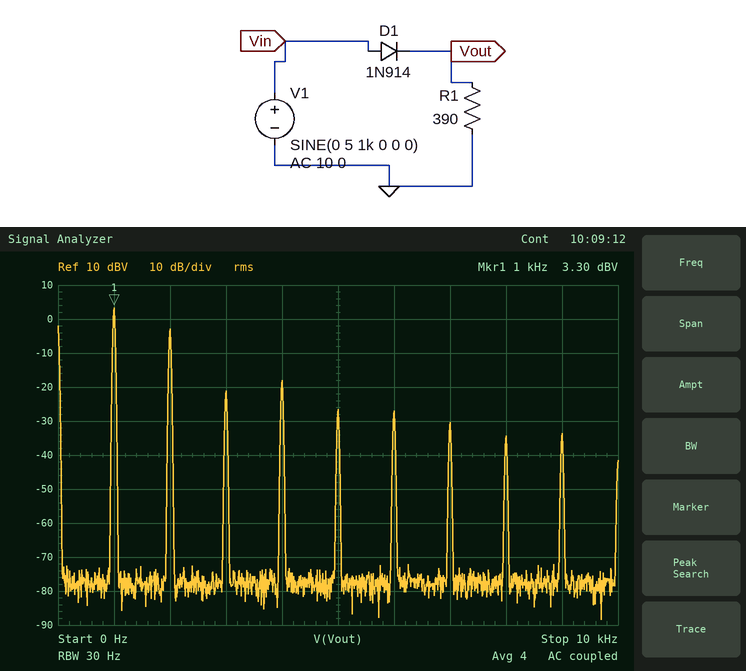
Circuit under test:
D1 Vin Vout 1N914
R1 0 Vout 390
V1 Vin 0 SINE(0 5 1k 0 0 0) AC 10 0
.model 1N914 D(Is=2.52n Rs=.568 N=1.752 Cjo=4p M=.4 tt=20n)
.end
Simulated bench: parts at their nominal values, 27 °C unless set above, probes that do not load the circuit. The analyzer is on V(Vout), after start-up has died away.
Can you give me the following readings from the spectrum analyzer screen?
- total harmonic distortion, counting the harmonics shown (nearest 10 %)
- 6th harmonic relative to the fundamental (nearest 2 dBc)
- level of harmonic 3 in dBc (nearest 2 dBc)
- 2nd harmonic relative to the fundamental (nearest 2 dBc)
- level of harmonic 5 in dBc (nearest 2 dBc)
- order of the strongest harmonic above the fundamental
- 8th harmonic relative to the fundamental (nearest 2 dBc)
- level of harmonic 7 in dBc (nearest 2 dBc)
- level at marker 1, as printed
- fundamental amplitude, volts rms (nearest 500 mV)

50 %
-30 dBc
-24 dBc
-6 dBc
-30 dBc
2
-38 dBc
-34 dBc
3.30 dBV
1.5 V
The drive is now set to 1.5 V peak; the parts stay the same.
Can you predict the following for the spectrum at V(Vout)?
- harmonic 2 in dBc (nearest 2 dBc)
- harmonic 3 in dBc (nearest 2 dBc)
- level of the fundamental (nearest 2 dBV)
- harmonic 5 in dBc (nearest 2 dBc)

-4 dBc
-14 dBc
-12 dBV
-22 dBc
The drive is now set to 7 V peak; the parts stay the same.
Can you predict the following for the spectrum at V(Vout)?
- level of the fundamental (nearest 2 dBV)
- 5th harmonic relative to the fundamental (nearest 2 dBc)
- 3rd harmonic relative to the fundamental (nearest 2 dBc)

6 dBV
-32 dBc
-28 dBc
